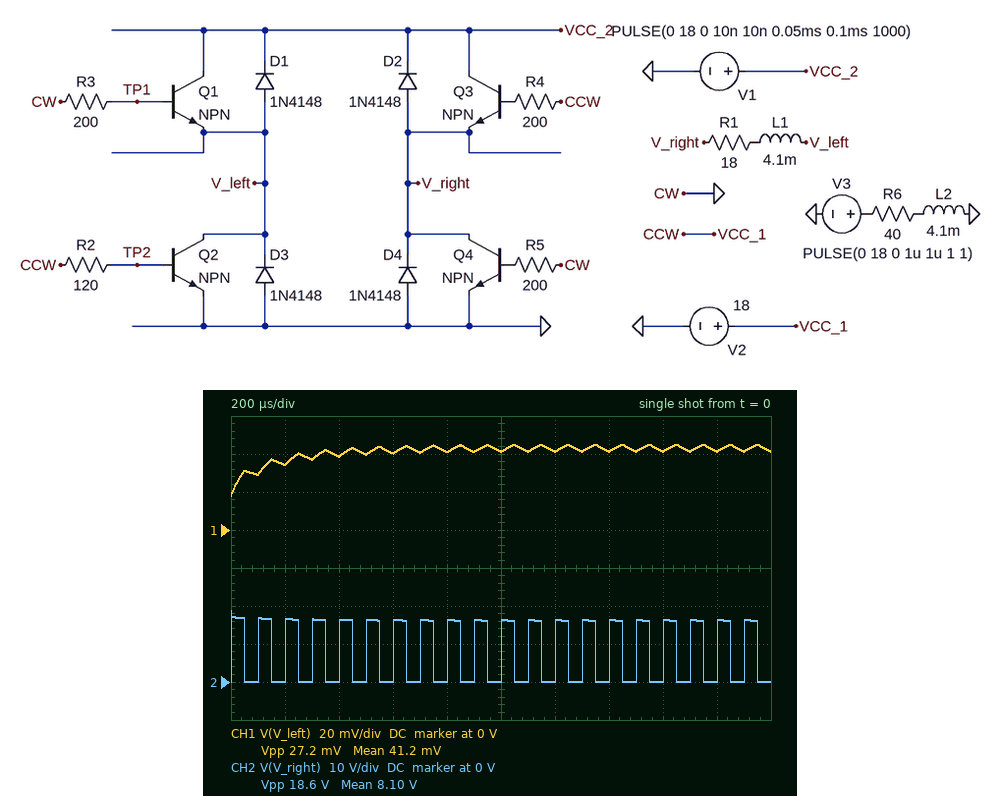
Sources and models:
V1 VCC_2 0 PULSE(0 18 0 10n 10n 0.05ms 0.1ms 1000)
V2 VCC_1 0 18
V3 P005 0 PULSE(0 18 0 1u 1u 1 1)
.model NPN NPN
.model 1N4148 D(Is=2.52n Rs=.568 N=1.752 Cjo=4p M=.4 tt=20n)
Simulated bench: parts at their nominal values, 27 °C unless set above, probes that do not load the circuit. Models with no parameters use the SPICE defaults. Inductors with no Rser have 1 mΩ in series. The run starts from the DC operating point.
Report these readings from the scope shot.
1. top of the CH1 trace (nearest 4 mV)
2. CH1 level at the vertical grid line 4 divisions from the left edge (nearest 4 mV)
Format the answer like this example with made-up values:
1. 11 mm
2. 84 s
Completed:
1. 44 mV
2. 40 mV
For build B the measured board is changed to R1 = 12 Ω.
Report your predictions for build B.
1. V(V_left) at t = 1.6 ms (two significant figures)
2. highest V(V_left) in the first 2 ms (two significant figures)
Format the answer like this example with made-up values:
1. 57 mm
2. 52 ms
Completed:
1. 48 mV
2. 51 mV
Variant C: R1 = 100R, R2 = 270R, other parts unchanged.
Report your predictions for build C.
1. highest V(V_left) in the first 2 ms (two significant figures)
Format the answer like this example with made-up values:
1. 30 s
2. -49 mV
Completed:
1. 37 mV
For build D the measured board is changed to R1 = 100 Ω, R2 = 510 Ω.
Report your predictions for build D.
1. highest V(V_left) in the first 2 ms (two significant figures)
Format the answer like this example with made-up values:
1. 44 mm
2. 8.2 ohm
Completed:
1. 47 mV
